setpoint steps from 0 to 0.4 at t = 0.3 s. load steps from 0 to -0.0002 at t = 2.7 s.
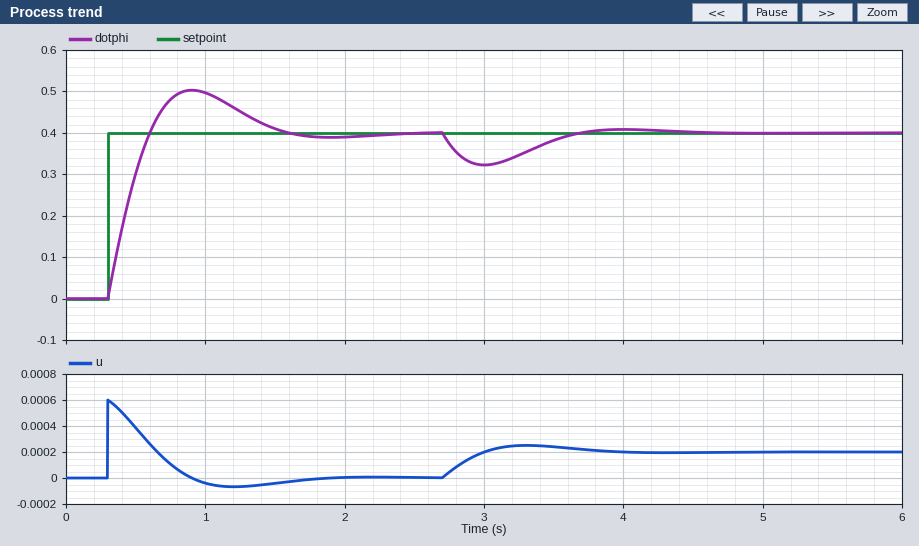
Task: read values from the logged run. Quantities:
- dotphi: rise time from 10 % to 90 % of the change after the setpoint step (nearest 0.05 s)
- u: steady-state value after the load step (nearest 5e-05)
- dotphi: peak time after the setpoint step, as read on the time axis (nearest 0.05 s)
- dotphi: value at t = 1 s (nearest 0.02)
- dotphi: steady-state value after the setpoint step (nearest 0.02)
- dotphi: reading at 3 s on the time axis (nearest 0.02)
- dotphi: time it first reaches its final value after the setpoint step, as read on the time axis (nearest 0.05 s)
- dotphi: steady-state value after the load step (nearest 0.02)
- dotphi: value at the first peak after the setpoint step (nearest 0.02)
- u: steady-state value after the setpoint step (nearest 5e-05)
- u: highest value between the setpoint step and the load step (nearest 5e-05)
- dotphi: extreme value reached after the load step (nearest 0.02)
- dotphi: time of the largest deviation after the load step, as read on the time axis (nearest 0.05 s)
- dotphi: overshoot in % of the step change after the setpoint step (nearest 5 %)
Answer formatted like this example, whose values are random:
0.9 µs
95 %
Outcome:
0.25 s
0.00020
0.90 s
0.50
0.40
0.32
0.60 s
0.40
0.50
0.00000
0.00060
0.32
3.00 s
25 %
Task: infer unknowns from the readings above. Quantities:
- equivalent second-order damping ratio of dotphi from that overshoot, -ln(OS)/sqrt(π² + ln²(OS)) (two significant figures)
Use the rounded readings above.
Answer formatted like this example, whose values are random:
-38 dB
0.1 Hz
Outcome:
0.40
